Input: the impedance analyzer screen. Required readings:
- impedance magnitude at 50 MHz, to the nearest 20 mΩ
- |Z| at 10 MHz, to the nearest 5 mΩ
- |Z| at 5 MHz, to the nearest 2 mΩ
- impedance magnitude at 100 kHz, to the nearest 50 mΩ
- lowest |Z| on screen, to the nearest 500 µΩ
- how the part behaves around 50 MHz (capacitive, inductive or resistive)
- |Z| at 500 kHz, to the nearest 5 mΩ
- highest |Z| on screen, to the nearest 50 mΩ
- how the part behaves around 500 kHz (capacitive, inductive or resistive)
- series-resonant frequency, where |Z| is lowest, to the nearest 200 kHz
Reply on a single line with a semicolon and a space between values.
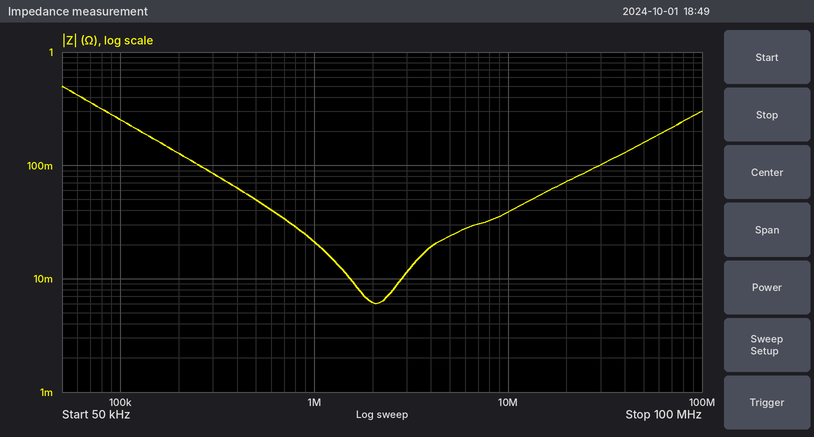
160 mΩ; 40 mΩ; 24 mΩ; 250 mΩ; 6.0 mΩ; inductive; 50 mΩ; 500 mΩ; capacitive; 2.0 MHz
